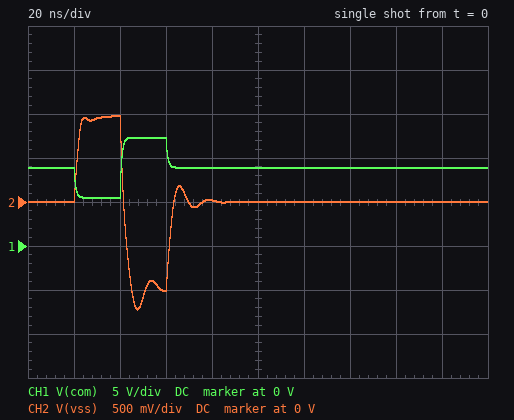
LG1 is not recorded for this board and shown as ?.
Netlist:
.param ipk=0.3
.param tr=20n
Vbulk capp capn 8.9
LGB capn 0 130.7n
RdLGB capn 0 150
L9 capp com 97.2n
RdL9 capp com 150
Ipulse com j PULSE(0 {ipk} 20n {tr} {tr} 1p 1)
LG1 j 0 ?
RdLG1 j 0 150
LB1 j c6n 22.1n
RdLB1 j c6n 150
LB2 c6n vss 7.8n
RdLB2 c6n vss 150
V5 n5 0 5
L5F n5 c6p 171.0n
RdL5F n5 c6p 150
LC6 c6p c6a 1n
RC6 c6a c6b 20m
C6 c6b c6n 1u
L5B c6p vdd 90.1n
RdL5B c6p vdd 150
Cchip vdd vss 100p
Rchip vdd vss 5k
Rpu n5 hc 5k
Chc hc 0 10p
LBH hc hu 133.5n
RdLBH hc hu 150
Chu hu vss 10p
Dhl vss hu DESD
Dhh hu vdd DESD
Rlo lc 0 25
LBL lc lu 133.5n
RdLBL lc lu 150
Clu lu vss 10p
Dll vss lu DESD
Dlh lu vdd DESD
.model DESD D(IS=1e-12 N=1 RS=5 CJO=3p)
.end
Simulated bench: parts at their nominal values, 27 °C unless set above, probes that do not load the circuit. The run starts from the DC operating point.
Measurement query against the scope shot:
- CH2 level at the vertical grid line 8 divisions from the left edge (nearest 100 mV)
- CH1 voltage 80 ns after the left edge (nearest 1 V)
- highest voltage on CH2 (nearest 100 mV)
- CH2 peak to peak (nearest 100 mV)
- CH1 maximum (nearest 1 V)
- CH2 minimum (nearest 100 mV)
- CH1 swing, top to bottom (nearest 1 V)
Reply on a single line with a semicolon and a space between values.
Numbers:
0 V; 9 V; 1.0 V; 2.2 V; 12 V; -1.2 V; 7 V
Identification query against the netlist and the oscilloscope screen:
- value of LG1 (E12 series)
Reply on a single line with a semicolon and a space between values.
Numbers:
120 nH
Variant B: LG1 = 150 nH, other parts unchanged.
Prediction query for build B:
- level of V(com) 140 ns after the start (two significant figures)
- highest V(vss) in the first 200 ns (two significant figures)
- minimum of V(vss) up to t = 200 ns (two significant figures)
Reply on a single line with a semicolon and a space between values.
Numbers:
8.9 V; 1.1 V; -1.4 V
